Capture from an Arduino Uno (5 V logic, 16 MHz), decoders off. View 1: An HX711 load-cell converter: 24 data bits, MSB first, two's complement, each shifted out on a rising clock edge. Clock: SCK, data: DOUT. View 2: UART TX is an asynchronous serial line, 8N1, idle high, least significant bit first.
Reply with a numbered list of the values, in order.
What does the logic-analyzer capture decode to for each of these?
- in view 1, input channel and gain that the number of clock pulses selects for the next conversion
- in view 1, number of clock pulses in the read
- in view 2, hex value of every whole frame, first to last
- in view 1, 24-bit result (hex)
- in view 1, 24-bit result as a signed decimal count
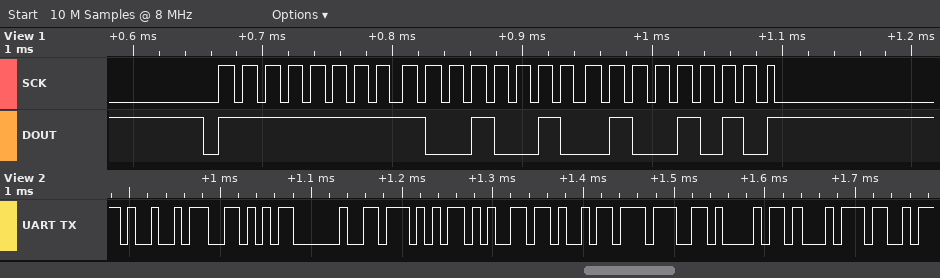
1. channel A, gain 128
2. 25
3. 0x49 0x56 0x20 0x57 0x65 0x69 0x67 0x68 0x74
4. 0xFF924A
5. -28086
